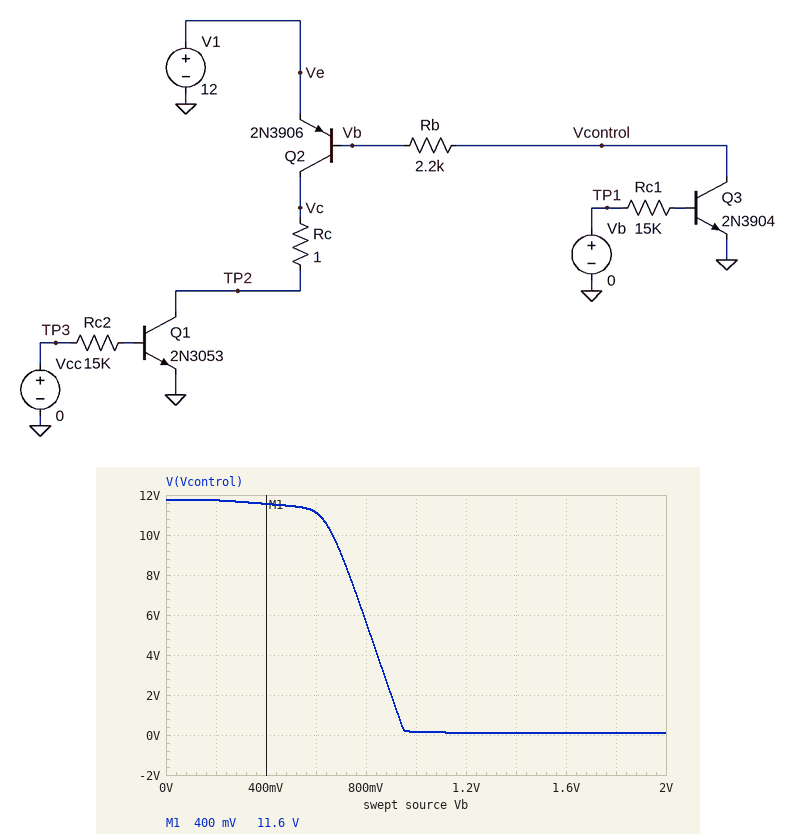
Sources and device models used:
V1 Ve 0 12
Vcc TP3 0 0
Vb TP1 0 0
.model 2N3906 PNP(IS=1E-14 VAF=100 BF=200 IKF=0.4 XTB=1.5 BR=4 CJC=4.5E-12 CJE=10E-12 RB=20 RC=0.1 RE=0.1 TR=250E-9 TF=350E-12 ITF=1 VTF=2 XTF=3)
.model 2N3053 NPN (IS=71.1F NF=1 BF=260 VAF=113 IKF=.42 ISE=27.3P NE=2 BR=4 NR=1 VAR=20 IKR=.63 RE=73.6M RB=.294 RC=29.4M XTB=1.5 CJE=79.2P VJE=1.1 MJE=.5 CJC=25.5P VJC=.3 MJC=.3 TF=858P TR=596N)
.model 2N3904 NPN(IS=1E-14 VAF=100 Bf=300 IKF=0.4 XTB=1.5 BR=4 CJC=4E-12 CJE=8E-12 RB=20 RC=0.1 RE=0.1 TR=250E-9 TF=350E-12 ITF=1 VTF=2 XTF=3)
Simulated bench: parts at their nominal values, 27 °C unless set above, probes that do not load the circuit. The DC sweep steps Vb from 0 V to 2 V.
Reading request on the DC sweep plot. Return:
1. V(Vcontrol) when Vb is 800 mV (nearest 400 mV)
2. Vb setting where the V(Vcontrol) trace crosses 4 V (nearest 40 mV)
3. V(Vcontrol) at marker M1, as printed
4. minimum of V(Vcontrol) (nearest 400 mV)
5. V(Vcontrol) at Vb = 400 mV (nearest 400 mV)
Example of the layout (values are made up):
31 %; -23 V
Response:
5.6 V; 840 mV; 11.6 V; 0 V; 11.6 V
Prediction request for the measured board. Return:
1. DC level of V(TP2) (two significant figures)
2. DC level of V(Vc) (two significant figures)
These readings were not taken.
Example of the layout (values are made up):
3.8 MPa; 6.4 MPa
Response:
12 V; 12 V
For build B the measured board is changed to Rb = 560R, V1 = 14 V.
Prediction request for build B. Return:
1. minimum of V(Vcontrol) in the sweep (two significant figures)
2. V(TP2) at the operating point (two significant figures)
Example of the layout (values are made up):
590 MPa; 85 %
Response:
190 mV; 14 V
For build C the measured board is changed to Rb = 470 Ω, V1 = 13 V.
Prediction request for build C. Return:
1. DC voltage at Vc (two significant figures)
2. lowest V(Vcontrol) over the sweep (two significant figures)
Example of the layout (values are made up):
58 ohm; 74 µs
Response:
13 V; 600 mV
